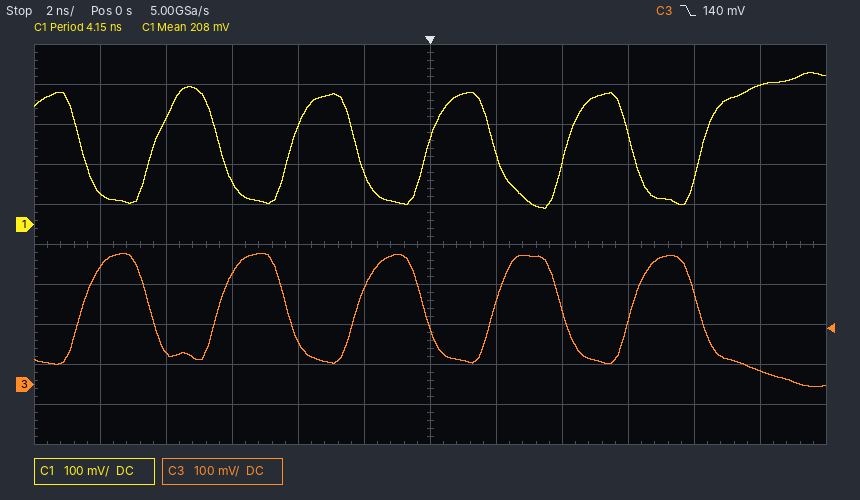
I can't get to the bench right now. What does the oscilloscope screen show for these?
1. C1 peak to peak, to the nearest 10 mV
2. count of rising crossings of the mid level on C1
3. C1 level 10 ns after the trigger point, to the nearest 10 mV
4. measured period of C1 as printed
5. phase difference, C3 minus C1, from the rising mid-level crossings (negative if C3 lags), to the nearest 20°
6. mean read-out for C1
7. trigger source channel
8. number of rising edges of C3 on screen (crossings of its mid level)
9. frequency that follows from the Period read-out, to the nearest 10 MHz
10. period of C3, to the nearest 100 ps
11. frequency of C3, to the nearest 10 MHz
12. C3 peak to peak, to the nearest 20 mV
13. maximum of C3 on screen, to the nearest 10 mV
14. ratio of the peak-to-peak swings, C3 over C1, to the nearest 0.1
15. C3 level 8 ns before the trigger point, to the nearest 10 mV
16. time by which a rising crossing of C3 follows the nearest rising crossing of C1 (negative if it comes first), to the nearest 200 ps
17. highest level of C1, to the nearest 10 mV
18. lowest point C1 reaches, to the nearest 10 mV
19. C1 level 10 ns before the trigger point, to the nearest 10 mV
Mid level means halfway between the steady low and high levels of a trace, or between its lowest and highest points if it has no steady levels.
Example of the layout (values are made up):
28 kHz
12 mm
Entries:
340 mV
5
350 mV
4.15 ns
-160°
208 mV
C3
5
240 MHz
4.2 ns
240 MHz
340 mV
330 mV
1.0
80 mV
+1.8 ns
380 mV
40 mV
80 mV
